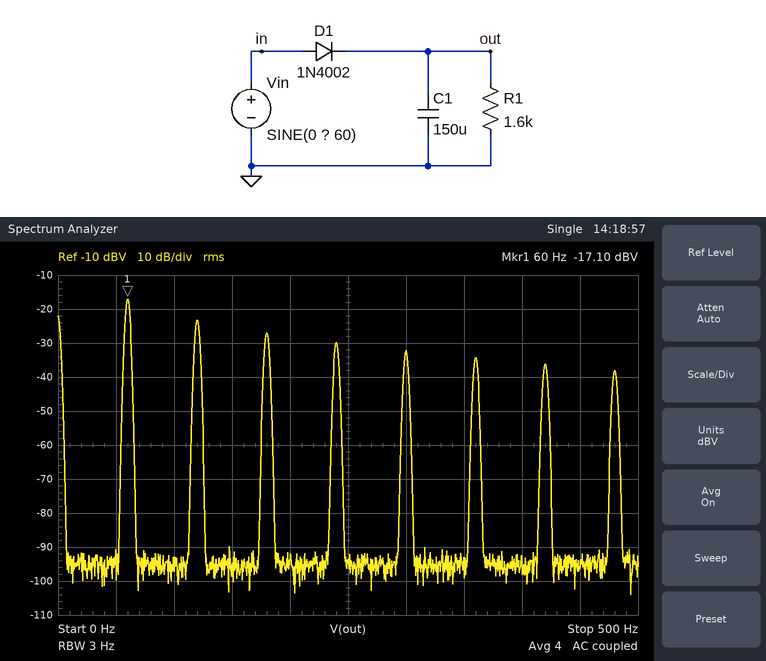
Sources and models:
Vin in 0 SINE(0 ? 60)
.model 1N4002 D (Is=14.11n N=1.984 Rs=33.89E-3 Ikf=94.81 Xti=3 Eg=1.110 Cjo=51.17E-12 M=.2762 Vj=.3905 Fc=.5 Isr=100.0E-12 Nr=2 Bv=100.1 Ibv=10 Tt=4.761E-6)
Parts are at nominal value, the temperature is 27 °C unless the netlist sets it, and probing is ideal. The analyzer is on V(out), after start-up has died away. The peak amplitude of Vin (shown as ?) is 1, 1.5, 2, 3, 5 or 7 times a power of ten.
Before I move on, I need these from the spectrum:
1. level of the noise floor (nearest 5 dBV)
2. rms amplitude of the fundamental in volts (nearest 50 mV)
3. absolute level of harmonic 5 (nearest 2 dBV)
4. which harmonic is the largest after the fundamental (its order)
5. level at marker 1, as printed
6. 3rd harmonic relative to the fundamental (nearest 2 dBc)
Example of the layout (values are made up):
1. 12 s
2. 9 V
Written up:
1. -95 dBV
2. 150 mV
3. -32 dBV
4. 2
5. -17.10 dBV
6. -10 dBc
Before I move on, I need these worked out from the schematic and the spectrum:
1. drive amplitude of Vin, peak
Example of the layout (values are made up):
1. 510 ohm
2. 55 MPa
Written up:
1. 10 V
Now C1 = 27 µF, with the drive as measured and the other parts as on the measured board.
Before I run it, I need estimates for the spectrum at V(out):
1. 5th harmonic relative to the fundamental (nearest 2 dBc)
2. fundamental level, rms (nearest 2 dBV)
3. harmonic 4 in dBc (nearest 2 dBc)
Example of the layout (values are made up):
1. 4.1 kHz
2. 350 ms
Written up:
1. -18 dBc
2. -4 dBV
3. -14 dBc
